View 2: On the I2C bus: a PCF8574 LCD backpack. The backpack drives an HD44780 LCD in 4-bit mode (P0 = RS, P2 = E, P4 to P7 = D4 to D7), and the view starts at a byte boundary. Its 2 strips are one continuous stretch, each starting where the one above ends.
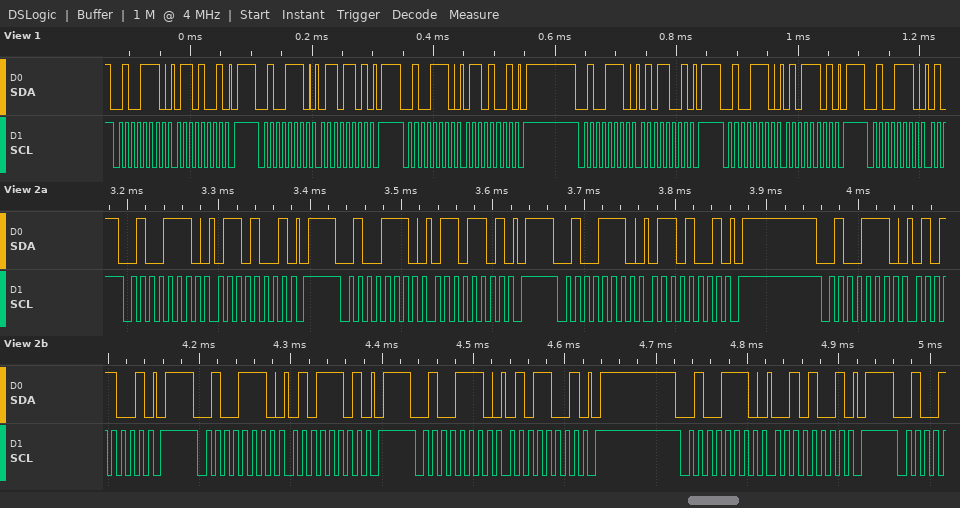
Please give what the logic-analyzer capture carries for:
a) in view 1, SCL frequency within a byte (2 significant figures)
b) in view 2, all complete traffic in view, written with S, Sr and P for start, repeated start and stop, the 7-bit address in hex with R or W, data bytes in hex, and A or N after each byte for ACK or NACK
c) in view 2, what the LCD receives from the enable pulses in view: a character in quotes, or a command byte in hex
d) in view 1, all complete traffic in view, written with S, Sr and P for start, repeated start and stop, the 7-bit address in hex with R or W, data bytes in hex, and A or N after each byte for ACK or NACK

100 kHz
S 27W A 69 A P S 27W A 6D A P S 27W A 69 A P S 27W A 59 A P S 27W A 5D A P S 27W A 59 A P S 27W A 29 A P
'e'
S 27W A 69 A P S 27W A 6D A P S 27W A 69 A P S 27W A 59 A P S 27W A 5D A P S 27W A
